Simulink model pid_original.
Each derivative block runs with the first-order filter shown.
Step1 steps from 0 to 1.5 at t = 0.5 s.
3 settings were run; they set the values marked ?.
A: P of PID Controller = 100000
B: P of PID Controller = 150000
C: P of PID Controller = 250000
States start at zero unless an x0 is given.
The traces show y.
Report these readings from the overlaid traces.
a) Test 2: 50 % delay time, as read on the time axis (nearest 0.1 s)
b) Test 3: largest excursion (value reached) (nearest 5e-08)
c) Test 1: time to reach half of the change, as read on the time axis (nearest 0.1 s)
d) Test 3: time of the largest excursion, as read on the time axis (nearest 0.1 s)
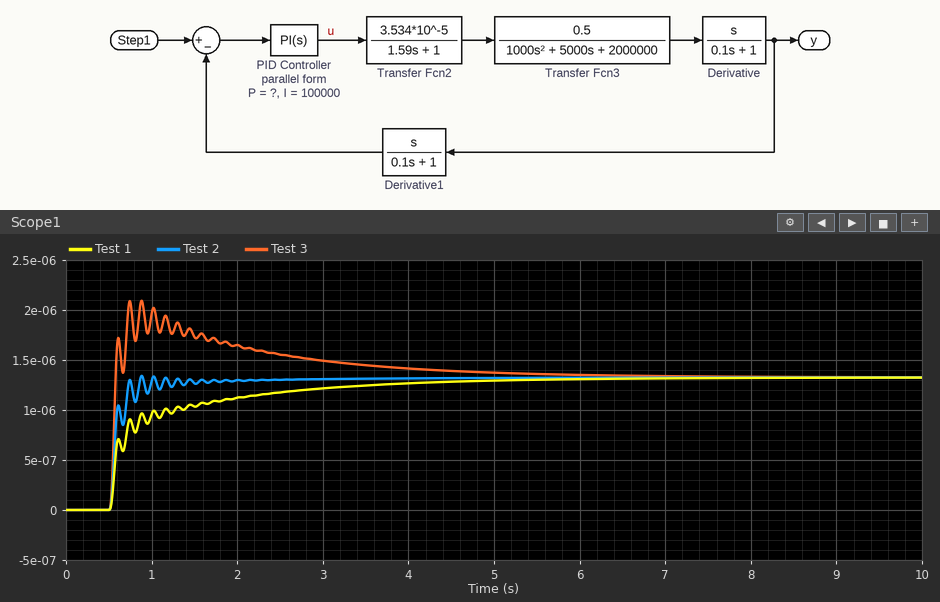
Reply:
0.6 s
0.00000210
0.6 s
0.9 s
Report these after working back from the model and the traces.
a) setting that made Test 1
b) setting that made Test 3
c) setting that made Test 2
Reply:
A
C
B
